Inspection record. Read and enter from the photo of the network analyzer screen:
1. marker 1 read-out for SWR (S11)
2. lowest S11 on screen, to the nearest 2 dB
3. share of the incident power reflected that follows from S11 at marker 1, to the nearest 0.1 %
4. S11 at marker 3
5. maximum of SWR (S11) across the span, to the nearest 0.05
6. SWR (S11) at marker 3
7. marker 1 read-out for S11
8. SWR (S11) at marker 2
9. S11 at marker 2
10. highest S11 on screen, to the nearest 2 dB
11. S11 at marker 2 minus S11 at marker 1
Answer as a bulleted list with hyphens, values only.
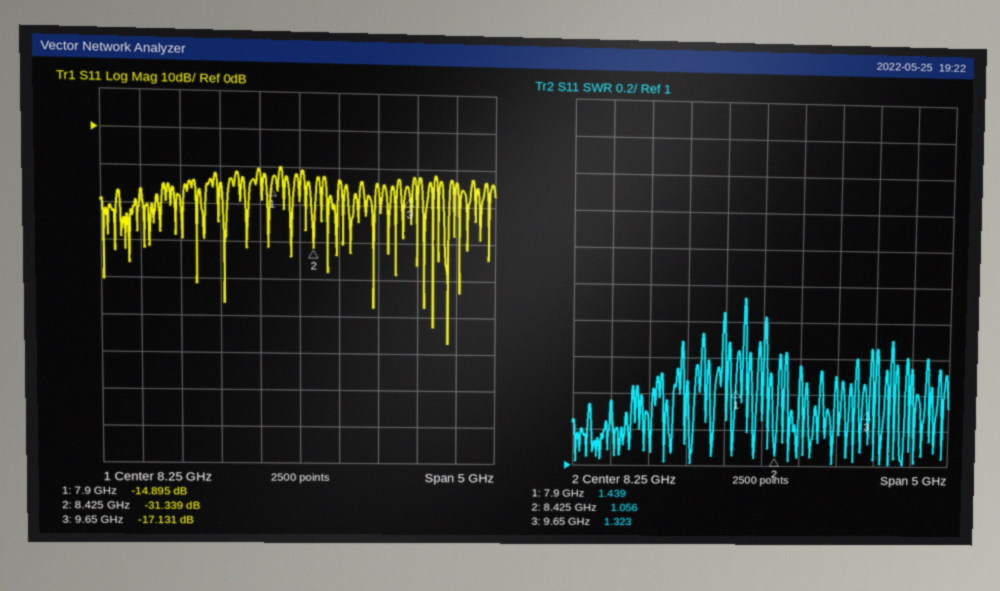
- 1.439
- -58 dB
- 3.2 %
- -17.131 dB
- 1.95
- 1.323
- -14.895 dB
- 1.056
- -31.339 dB
- -10 dB
- -16.444 dB
